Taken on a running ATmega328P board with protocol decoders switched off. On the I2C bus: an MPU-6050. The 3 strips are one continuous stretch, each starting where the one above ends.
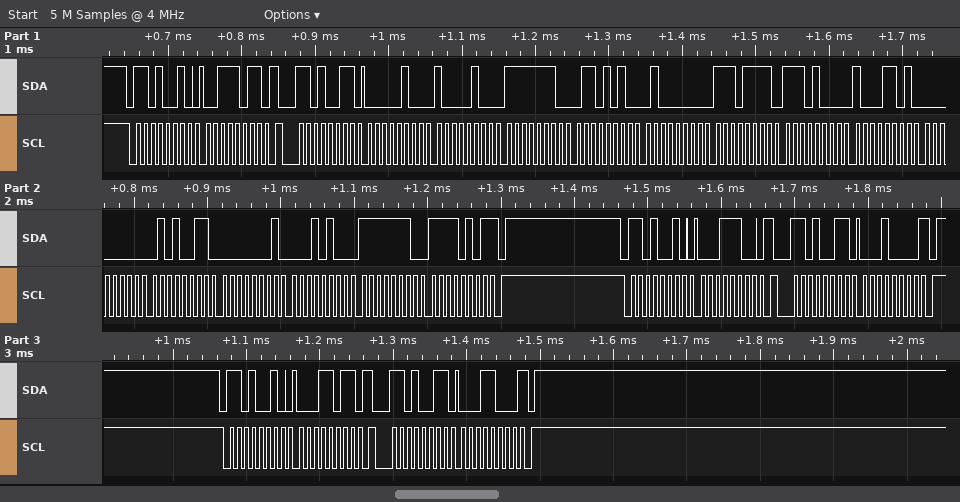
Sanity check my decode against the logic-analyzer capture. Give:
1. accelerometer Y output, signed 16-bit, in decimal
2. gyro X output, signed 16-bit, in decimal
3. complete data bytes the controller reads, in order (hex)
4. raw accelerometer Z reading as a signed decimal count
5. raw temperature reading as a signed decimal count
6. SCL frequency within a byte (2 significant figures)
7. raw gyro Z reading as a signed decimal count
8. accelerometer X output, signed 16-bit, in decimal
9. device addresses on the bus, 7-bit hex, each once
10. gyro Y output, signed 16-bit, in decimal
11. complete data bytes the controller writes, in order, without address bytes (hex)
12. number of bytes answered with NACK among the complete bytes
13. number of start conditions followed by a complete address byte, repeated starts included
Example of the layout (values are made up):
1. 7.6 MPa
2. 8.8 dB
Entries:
1. -406
2. 83
3. 04 84 FE 6A 40 EF E8 8D 00 53 01 14 FE F5 10 18
4. 16623
5. -6003
6. 100 kHz
7. -267
8. 1156
9. 0x69
10. 276
11. 3B 1C 1B
12. 3
13. 6
